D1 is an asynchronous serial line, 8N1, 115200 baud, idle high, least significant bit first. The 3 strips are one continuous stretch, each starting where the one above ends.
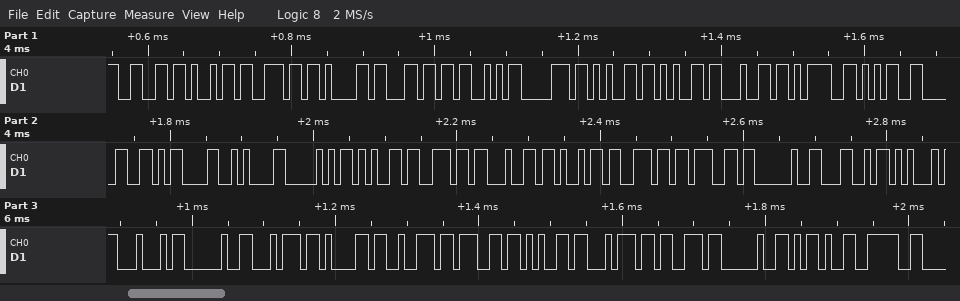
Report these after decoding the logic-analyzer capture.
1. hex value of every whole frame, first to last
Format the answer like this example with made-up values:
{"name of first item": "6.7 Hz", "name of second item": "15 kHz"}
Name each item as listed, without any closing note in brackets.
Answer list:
{"hex value of every whole frame, first to last": "66 69 6E 61 6C 53 70 65 65 64 3D 35 30 0D 0A 50 65 6E 64 69 6E 67 20 4C 45 44 20 74 61 72 67 65 74 73 20 2D 3E"}
